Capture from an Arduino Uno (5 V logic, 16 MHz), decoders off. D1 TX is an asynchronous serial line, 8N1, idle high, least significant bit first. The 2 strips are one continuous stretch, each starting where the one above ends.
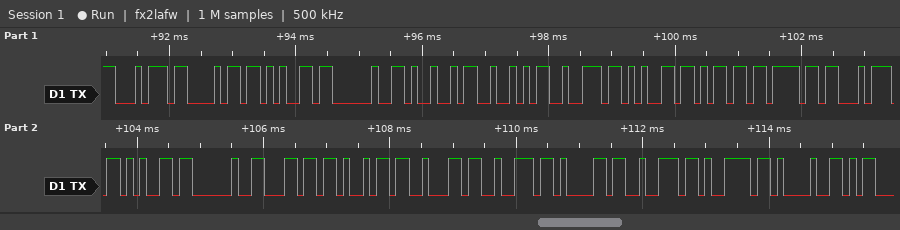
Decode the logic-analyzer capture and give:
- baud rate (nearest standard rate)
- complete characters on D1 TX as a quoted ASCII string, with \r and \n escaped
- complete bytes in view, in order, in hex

9600 baud
"the IRremote library!"
74 68 65 20 49 52 72 65 6D 6F 74 65 20 6C 69 62 72 61 72 79 21
